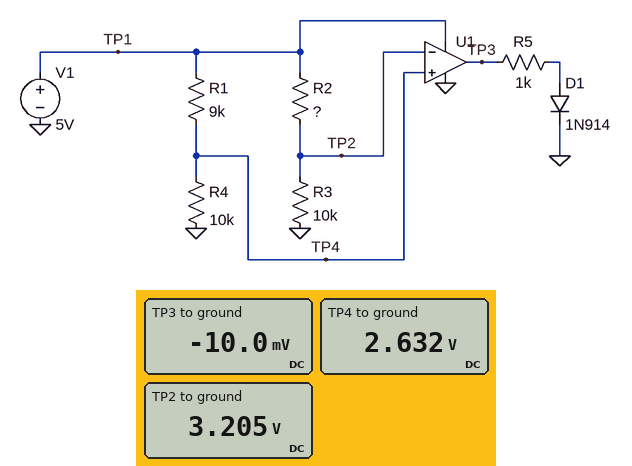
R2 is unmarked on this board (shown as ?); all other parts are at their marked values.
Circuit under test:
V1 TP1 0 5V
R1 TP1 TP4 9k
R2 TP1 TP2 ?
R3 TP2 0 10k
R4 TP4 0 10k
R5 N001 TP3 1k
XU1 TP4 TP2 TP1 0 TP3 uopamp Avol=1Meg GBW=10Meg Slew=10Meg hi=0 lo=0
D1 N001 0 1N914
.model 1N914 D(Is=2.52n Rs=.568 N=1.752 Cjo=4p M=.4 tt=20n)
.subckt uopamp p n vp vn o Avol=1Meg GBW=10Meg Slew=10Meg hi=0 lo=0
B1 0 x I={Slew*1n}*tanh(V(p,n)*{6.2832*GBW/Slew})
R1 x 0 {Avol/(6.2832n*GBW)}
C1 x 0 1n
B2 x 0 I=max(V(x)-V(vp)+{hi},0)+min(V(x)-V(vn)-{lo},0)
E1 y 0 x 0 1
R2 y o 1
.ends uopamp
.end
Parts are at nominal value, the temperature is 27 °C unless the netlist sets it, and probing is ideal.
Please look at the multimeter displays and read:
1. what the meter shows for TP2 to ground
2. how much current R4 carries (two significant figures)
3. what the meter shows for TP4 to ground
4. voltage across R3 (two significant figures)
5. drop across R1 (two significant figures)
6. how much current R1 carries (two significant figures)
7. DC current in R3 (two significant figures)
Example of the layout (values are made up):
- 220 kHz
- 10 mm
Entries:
- 3.205 V
- 260 µA
- 2.632 V
- 3.2 V
- 2.4 V
- 260 µA
- 320 µA
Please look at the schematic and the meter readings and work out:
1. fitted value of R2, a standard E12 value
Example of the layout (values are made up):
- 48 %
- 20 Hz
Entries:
- 5.6 kΩ
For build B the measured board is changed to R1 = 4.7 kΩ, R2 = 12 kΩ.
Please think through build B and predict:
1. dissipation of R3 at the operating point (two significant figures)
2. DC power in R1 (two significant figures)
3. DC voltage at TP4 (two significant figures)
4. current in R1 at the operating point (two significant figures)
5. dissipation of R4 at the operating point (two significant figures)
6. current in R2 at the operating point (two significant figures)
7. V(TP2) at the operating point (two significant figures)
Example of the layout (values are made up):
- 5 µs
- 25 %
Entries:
- 520 µW
- 540 µW
- 3.4 V
- 340 µA
- 1.2 mW
- 230 µA
- 2.3 V
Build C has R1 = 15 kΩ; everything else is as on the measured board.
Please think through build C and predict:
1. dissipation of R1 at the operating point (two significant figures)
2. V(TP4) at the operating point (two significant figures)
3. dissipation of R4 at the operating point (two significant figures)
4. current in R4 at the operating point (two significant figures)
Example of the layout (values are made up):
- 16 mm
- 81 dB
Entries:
- 600 µW
- 2.0 V
- 400 µW
- 200 µA
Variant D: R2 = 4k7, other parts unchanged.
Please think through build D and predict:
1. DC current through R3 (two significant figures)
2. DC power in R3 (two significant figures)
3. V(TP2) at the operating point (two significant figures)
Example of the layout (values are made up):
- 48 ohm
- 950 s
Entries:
- 340 µA
- 1.2 mW
- 3.4 V
